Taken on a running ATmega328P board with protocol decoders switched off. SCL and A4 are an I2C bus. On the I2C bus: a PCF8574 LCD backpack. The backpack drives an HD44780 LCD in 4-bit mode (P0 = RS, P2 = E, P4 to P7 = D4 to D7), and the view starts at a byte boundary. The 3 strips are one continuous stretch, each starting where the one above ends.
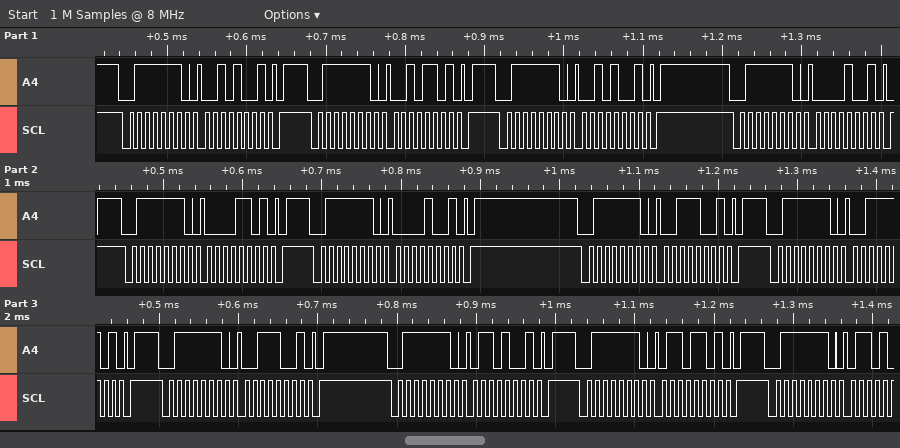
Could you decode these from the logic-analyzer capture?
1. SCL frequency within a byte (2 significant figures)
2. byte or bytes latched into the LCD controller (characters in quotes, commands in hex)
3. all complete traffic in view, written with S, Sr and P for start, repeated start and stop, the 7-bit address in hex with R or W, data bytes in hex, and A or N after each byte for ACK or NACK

100 kHz
' '
S 3FW A 29 A P S 3FW A 2D A P S 3FW A 29 A P S 3FW A 09 A P S 3FW A 0D A P S 3FW A 09 A P S 3FW A 39 A P S 3FW A 3D A P S 3FW A 39 A P S 3FW A 69 A P S 3FW A 6D A P S 3FW A
